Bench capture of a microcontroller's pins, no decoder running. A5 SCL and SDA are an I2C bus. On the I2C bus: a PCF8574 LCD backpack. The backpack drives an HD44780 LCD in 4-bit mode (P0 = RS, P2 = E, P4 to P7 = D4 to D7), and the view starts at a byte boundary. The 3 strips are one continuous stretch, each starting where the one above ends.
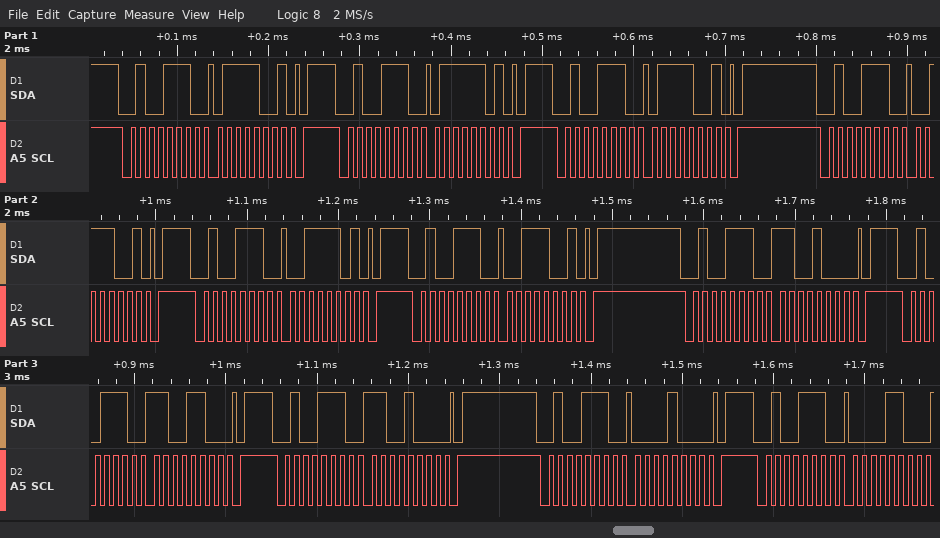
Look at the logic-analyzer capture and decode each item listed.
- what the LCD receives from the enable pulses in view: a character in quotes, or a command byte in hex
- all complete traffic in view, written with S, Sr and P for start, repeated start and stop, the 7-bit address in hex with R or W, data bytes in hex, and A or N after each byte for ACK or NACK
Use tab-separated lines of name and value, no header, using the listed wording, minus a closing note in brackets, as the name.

what the LCD receives from the enable pulses in view: a character in quotes, or a command byte in hex	's'
all complete traffic in view, written with S, Sr and P for start, repeated start and stop, the 7-bit address in hex with R or W, data bytes in hex, and A or N after each byte for ACK or NACK	S 27W A 79 A P S 27W A 7D A P S 27W A 79 A P S 27W A 39 A P S 27W A 3D A P S 27W A 39 A P S 27W A C8 A P S 27W A CC A P S 27W A C8 A P S 27W A 08 A P S 27W A 0C A
